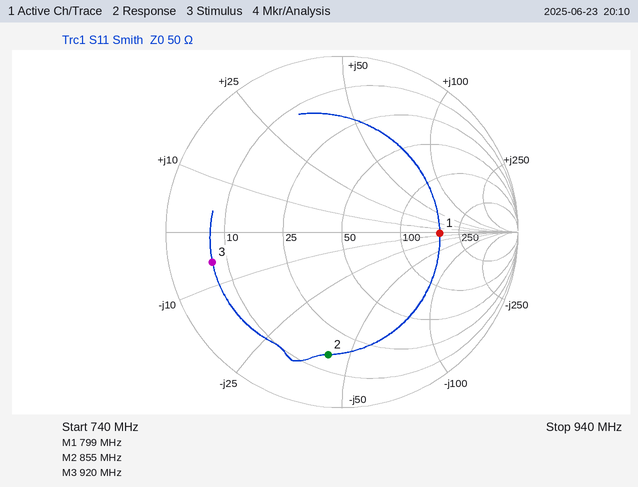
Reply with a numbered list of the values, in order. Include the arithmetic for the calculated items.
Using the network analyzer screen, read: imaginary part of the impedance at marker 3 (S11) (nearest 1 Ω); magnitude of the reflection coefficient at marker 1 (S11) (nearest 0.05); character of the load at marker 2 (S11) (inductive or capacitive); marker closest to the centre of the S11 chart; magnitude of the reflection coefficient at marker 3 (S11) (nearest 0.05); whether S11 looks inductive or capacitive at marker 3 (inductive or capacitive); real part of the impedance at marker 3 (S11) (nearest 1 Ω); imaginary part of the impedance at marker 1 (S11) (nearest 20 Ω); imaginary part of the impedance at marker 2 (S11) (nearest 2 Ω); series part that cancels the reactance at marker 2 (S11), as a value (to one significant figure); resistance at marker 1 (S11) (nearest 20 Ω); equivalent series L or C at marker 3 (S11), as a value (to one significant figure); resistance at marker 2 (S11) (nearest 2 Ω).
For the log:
1. -6 Ω
2. 0.55
3. capacitive
4. marker 1
5. 0.75
6. capacitive
7. 7 Ω
8. 0 Ω
9. -42 Ω
10. L = 42 Ω/(2π × 855 MHz) ≈ 8 nH
11. 180 Ω
12. C = 1/(2π × 920 MHz × 6 Ω) ≈ 28.8 pF, so 30 pF to one significant figure
13. 16 Ω
